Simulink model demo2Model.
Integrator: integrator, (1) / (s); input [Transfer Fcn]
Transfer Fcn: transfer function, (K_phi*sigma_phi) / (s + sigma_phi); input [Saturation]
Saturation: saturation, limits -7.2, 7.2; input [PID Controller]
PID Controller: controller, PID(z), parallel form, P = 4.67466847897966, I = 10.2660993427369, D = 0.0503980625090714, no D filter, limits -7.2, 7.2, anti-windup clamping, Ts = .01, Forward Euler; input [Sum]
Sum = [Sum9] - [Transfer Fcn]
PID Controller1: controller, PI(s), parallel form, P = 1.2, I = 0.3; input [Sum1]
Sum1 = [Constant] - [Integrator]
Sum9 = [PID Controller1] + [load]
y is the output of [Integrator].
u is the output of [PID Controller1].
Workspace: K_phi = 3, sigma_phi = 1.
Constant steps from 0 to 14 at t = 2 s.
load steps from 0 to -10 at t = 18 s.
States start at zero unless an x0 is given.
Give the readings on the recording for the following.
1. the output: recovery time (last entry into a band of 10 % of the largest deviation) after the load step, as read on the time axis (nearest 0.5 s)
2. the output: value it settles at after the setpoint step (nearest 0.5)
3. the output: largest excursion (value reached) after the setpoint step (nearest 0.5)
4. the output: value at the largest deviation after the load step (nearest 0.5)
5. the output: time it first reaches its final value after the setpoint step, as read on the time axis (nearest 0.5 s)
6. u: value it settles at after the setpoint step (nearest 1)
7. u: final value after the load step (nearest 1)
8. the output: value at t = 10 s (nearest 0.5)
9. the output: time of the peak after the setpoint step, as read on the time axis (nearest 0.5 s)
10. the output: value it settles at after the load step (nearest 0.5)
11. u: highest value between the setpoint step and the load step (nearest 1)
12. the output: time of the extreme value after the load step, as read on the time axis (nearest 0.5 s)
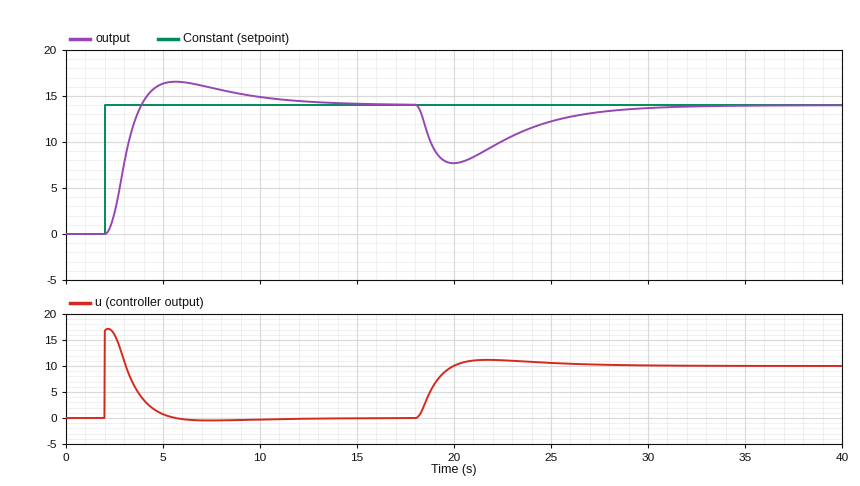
28.0 s
14.0
16.5
7.5
4.0 s
0
10
15.0
5.5 s
14.0
17
20.0 s
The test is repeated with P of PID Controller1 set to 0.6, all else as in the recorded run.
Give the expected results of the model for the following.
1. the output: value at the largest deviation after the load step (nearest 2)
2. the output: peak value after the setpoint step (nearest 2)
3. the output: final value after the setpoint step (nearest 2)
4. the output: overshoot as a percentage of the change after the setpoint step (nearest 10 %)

4
18
14
30 %
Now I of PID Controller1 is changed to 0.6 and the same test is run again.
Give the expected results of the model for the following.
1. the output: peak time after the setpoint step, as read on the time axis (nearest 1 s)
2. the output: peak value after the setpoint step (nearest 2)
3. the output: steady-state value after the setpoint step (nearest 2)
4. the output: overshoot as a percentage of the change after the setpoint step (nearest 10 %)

5 s
18
14
30 %
